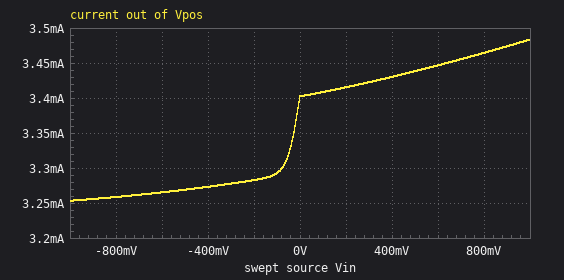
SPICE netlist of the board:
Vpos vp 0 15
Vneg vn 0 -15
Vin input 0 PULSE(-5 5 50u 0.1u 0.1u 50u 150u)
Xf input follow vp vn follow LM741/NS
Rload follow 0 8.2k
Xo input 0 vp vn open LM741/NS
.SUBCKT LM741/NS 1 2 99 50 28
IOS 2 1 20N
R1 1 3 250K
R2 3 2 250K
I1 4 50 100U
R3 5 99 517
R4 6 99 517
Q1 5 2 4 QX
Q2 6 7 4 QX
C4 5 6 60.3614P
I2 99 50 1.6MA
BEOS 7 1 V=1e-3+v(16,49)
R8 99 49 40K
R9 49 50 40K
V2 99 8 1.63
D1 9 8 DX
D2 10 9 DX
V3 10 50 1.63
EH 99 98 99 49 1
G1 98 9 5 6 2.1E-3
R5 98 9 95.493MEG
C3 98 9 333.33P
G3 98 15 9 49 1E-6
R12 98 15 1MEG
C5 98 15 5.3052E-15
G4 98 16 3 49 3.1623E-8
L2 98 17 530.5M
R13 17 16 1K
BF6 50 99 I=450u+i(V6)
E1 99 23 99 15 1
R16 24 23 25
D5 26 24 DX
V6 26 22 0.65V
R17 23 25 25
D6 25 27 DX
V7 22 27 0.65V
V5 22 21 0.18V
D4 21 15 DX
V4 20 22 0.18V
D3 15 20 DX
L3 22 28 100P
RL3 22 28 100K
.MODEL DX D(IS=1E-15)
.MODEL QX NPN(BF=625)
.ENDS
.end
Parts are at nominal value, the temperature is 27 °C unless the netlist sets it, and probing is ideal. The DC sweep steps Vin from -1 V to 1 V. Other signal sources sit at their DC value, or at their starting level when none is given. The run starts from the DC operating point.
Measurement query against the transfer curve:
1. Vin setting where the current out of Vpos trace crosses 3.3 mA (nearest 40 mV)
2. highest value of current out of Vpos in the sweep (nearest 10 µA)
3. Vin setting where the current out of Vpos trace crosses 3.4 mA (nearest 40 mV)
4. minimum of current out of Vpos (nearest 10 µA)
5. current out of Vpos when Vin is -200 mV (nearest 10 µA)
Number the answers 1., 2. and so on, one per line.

1. -80 mV
2. 3.48 mA
3. 0 V
4. 3.25 mA
5. 3.28 mA
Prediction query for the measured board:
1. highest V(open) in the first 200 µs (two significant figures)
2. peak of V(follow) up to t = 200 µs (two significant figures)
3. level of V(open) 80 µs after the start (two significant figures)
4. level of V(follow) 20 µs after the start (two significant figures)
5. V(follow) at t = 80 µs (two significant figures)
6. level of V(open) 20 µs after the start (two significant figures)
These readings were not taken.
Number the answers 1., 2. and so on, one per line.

1. 2.3 V
2. 5.0 V
3. -4.3 V
4. -5.0 V
5. 4.6 V
6. -14 V
